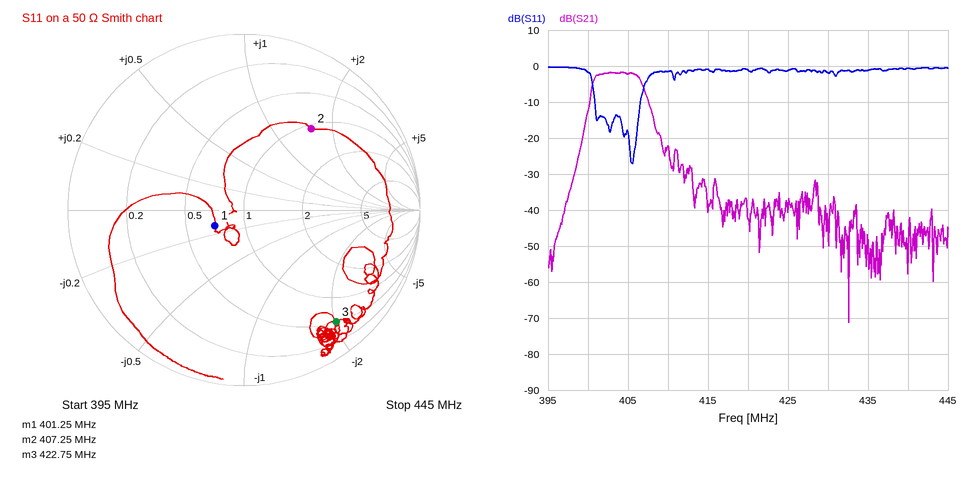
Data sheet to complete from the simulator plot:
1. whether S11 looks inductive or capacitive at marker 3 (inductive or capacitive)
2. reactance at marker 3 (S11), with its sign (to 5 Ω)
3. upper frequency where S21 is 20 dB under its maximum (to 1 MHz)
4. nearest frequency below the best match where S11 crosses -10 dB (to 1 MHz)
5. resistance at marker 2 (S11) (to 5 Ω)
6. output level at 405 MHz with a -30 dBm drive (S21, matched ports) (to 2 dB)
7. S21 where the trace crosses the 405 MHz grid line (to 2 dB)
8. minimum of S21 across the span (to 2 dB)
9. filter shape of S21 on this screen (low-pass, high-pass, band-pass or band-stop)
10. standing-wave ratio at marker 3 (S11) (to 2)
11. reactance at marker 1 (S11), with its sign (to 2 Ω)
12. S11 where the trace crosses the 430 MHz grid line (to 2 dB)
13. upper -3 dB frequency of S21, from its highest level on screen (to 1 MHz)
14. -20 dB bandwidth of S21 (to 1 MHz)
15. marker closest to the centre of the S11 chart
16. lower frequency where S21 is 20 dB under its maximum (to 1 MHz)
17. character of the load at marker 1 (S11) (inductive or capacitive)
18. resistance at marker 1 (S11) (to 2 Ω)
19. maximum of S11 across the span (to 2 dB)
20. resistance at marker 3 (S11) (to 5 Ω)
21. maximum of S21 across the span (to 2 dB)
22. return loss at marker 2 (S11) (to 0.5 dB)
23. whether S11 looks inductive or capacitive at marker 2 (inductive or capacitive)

capacitive
-100 Ω
409 MHz
401 MHz
55 Ω
-32 dBm
-2 dB
-72 dB
band-pass
10
-6 Ω
-2 dB
407 MHz
10 MHz
marker 1
399 MHz
capacitive
36 Ω
0 dB
25 Ω
-2 dB
4.5 dB
inductive
